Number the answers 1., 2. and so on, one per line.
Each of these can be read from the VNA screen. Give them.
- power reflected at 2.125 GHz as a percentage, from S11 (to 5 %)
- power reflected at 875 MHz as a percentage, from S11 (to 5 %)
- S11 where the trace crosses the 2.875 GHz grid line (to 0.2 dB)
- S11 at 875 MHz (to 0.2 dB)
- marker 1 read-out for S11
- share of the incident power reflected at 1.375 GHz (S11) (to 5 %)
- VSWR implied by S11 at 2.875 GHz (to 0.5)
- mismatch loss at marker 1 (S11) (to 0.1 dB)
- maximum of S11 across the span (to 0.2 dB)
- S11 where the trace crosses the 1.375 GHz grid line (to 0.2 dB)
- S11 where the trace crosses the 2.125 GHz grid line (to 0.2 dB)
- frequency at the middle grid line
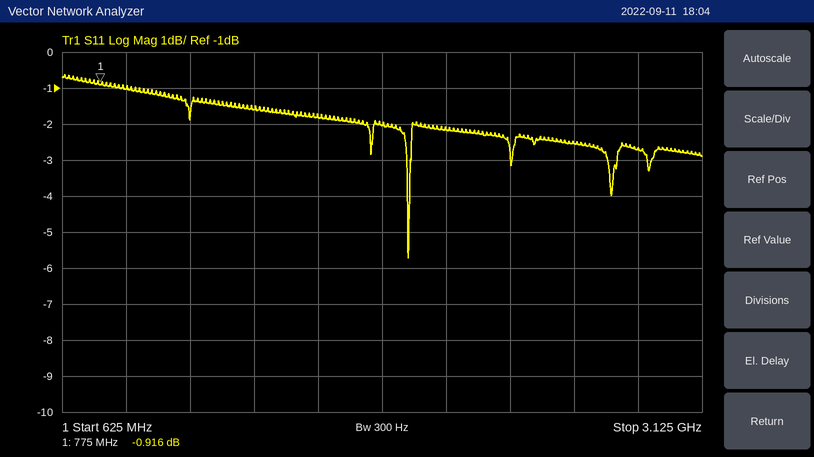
1. 60 %
2. 80 %
3. -2.6 dB
4. -1.0 dB
5. -0.916 dB
6. 70 %
7. 6.5
8. 7.2 dB
9. -0.6 dB
10. -1.6 dB
11. -2.2 dB
12. 1.875 GHz
